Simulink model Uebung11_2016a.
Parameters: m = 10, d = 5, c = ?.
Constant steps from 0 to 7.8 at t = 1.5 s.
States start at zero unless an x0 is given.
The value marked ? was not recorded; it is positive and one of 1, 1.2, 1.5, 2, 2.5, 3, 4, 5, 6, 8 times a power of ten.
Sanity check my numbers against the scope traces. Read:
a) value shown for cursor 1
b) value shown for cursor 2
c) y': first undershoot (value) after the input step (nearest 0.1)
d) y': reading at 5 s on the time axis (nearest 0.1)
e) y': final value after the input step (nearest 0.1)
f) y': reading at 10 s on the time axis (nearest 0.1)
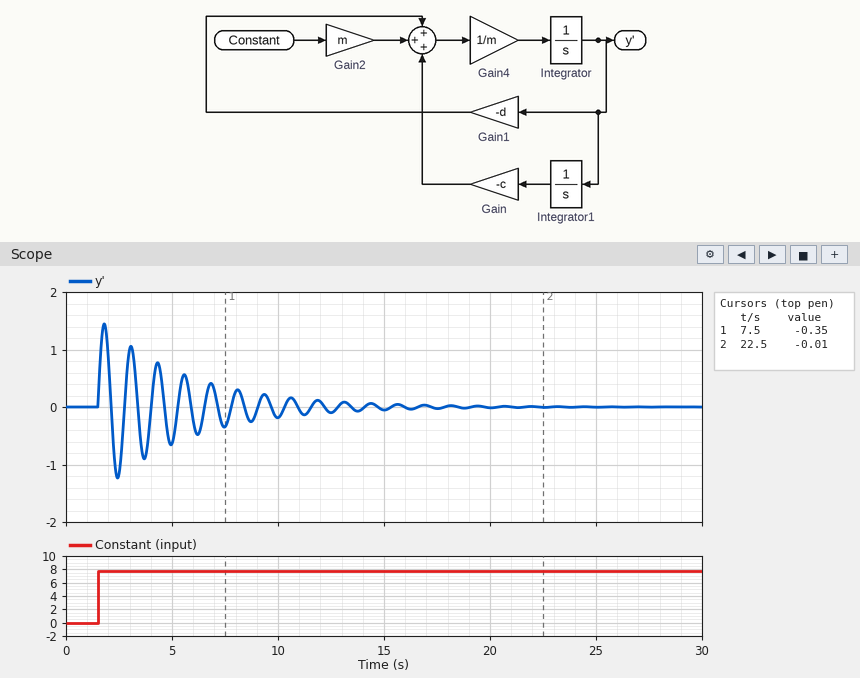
-0.35
-0.01
-1.2
-0.6
0.0
-0.2
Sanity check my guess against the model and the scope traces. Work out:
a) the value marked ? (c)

250
